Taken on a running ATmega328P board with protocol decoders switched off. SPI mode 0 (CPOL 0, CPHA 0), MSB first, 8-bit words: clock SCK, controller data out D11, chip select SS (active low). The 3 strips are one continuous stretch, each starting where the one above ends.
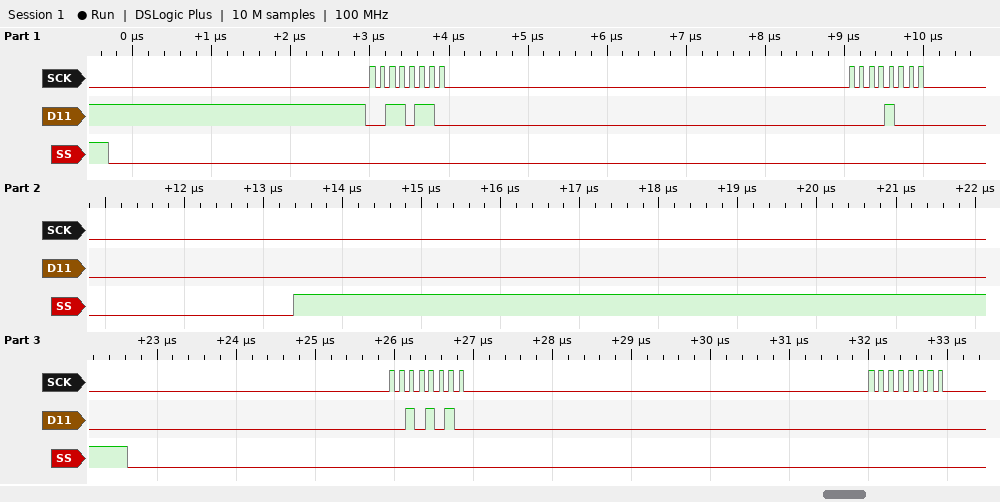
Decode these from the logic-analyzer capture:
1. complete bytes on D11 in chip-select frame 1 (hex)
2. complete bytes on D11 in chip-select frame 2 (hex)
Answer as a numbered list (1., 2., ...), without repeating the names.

1. 36 08
2. 2A 00
